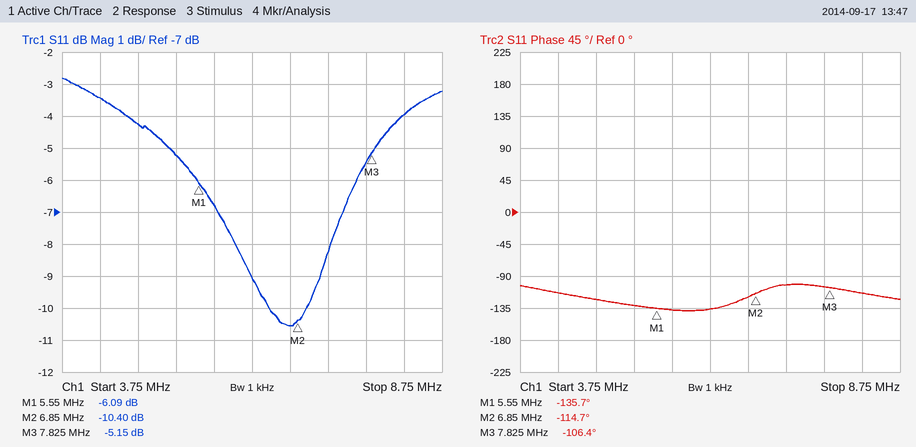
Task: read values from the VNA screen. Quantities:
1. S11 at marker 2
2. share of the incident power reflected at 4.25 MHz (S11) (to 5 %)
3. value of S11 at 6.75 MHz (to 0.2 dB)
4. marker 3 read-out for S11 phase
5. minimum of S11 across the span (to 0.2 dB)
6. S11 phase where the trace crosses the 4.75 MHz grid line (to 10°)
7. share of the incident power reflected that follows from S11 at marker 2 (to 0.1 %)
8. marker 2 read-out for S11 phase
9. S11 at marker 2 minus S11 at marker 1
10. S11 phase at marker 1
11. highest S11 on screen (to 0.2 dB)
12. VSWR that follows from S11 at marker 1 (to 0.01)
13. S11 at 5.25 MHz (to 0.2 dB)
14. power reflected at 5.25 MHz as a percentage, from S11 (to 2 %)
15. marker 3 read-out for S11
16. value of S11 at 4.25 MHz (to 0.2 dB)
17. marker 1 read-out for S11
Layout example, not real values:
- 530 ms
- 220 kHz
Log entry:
- -10.40 dB
- 45 %
- -10.6 dB
- -106.4°
- -10.6 dB
- -120°
- 9.1 %
- -114.7°
- -4.31 dB
- -135.7°
- -2.8 dB
- 2.97
- -5.2 dB
- 30 %
- -5.15 dB
- -3.4 dB
- -6.09 dB
